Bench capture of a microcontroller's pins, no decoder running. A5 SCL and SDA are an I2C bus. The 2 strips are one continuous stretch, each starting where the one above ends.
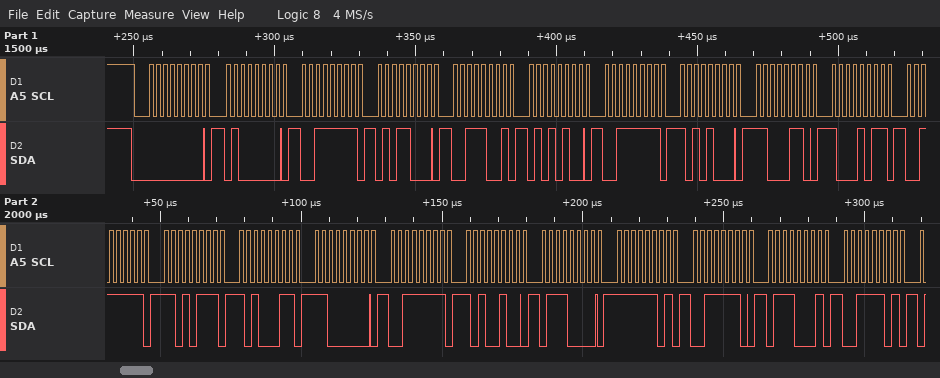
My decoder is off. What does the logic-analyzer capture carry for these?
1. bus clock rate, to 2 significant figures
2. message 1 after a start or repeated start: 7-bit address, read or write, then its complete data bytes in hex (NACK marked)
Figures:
400 kHz
0x00 write: 40 3F 58 39 54 3F A8 C6 8B 3F D7 A3 C0 3F A4 70 FD 3E 71 3D
